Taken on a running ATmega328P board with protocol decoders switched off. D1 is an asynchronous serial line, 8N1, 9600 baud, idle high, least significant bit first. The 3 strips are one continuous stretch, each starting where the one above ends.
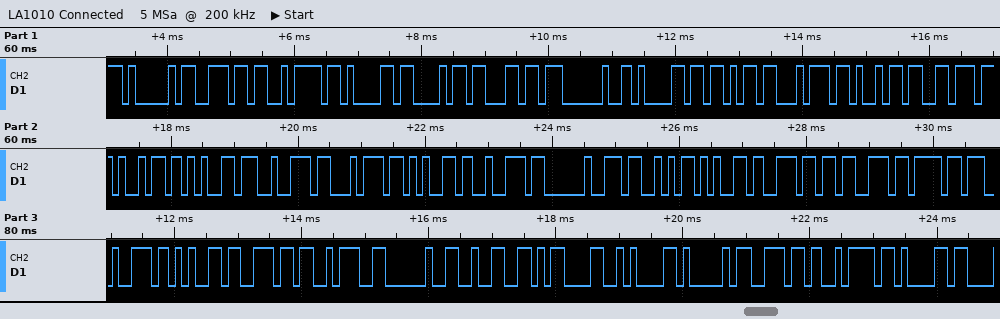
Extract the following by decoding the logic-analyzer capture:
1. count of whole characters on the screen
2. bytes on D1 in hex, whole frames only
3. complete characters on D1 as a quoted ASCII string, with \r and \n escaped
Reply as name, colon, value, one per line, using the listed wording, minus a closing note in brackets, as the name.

count of whole characters on the screen: 36
bytes on D1 in hex, whole frames only: 0x41 0x6E 0x7A 0x61 0x68 0x6C 0x20 0x61 0x6B 0x74 0x69 0x76 0x69 0x65 0x72 0x74 0x65 0x72 0x20 0x53 0x65 0x6E 0x73 0x6F 0x72 0x65 0x6E 0x3A 0x20 0x32 0x0D 0x0A 0x41 0x6E 0x7A 0x61
complete characters on D1 as a quoted ASCII string, with \r and \n escaped: "Anzahl aktivierter Sensoren: 2\r\nAnza"
